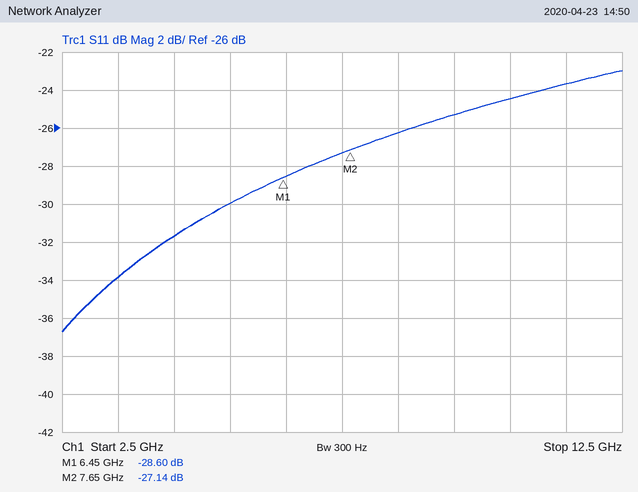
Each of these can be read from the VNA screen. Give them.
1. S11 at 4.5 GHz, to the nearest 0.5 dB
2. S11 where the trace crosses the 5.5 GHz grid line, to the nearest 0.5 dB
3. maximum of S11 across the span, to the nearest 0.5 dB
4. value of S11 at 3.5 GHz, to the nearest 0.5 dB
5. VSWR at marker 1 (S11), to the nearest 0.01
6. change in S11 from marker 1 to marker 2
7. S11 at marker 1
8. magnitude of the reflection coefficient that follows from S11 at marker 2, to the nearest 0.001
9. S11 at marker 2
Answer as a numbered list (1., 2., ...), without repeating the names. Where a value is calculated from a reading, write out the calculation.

1. -31.5 dB
2. -30.0 dB
3. -23.0 dB
4. -34.0 dB
5. (1 + 0.0372)/(1 − 0.0372) ≈ 1.08
6. -27.14 − (-28.6) = 1.46 dB
7. -28.60 dB
8. 10^(-27.14/20) ≈ 0.044
9. -27.14 dB
